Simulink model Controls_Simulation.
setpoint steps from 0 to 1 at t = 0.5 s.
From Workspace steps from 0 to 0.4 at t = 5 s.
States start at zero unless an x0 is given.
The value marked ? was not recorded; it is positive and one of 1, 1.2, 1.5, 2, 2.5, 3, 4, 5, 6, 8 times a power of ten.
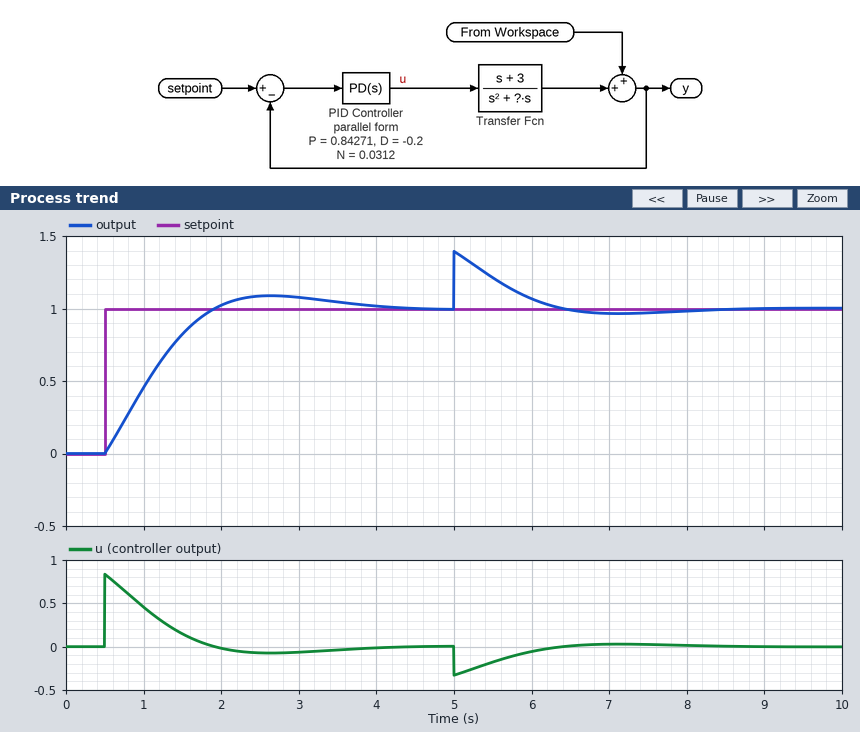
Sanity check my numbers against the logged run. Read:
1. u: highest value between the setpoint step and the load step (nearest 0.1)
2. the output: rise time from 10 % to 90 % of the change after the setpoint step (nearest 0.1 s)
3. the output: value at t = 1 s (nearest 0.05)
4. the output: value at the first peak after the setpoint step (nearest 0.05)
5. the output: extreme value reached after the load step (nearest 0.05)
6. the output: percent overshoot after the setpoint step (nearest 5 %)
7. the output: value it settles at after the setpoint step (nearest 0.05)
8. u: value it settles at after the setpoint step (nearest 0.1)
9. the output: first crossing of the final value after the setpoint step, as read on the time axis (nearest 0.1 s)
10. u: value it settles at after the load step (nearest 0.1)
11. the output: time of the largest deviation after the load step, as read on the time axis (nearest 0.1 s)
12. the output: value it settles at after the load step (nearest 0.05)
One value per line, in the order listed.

0.8
1.0 s
0.45
1.10
1.40
10 %
1.00
0.0
1.9 s
0.0
5.0 s
1.00
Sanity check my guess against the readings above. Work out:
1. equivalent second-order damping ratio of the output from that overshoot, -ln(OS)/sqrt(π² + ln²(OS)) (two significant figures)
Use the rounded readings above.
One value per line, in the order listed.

0.59
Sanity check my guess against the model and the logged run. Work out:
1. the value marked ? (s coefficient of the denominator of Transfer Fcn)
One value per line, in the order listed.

1.2
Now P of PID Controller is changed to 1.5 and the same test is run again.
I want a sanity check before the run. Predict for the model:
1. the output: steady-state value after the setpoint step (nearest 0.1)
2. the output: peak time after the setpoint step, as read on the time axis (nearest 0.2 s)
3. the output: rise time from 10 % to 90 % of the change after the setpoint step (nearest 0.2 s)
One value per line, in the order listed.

1.0
2.0 s
0.6 s
